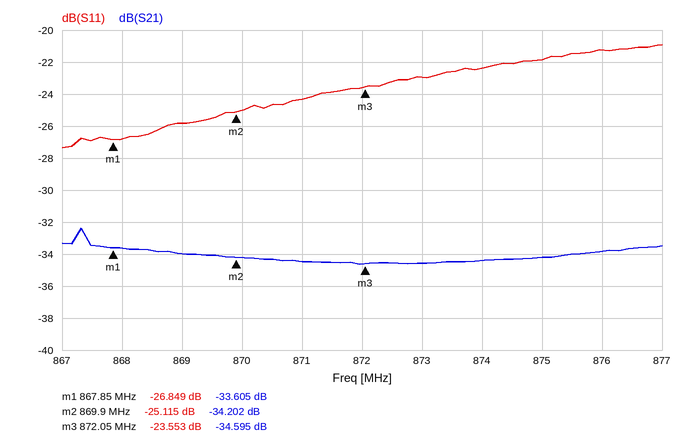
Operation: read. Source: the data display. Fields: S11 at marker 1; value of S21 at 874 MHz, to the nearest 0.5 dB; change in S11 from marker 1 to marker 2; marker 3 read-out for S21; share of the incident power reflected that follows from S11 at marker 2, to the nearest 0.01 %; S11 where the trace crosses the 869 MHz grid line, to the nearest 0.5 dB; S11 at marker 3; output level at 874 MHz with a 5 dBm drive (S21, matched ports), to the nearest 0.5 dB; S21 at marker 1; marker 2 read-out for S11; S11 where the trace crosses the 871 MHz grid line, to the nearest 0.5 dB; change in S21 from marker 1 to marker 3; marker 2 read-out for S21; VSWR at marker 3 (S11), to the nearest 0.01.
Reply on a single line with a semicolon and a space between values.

-26.849 dB; -34.5 dB; 1.734 dB; -34.595 dB; 0.31 %; -26.0 dB; -23.553 dB; -29.5 dBm; -33.605 dB; -25.115 dB; -24.5 dB; -0.990 dB; -34.202 dB; 1.14
